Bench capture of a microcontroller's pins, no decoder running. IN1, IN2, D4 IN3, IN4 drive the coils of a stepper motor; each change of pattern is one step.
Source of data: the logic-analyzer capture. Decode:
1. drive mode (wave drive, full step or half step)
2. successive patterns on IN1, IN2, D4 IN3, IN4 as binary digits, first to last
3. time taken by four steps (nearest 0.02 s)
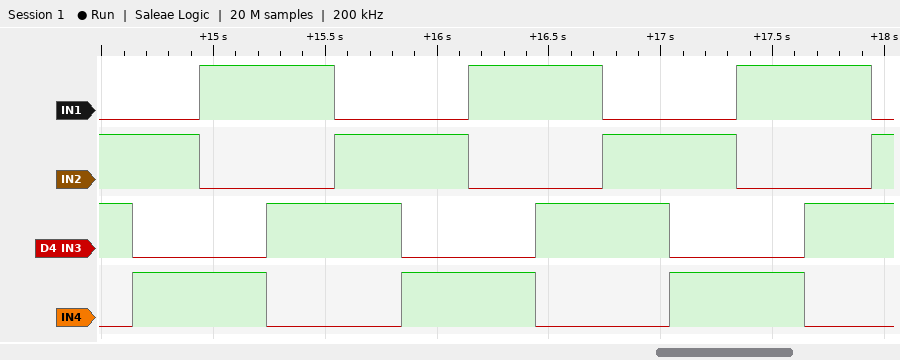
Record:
full step
0110 0101 1001 1010 0110 0101 1001 1010 0110 0101 1001 1010 0110
1.20 s
